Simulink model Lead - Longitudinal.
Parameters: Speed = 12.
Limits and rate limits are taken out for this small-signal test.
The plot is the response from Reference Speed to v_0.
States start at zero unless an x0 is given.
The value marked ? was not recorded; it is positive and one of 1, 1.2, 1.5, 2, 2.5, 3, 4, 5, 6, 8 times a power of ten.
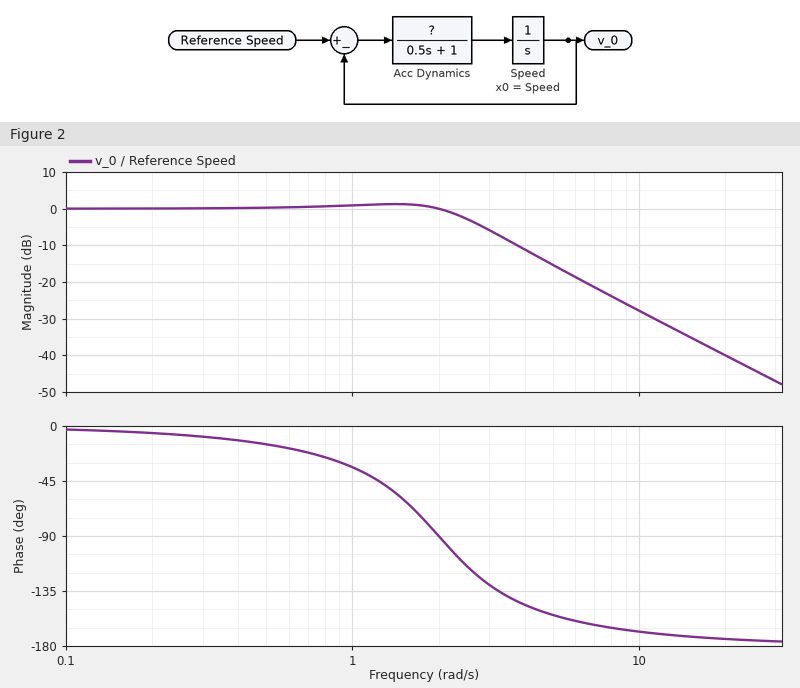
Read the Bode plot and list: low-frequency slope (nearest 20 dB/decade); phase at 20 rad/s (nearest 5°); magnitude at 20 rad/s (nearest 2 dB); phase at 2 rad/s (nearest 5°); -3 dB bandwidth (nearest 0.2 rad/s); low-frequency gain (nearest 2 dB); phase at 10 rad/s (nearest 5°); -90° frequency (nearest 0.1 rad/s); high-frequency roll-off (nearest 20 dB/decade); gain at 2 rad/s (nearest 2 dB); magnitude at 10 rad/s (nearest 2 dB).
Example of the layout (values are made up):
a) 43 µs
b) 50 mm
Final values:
a) 0 dB/decade
b) -175°
c) -40 dB
d) -90°
e) 2.6 rad/s
f) 0 dB
g) -170°
h) 2.0 rad/s
i) -40 dB/decade
j) 0 dB
k) -28 dB
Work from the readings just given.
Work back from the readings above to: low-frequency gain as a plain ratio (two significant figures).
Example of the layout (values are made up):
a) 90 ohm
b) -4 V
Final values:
a) 1.0
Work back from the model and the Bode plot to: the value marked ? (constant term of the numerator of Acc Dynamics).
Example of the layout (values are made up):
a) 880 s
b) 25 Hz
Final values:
a) 2
